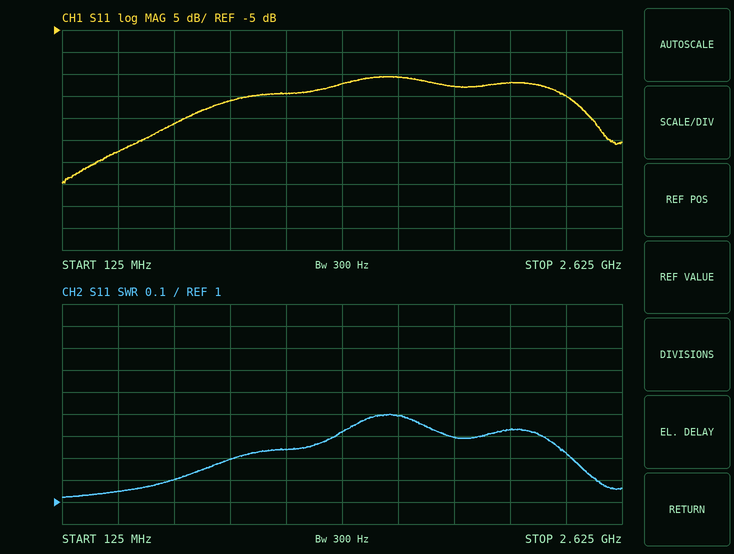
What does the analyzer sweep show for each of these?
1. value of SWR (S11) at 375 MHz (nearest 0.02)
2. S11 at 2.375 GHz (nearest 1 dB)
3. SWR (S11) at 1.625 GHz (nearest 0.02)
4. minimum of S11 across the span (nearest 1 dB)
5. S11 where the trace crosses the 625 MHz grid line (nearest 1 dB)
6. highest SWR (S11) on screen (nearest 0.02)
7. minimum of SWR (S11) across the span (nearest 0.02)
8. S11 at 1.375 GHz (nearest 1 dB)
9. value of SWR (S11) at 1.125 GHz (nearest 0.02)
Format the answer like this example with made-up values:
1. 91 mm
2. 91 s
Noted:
1. 1.04
2. -20 dB
3. 1.40
4. -40 dB
5. -26 dB
6. 1.40
7. 1.02
8. -17 dB
9. 1.24
